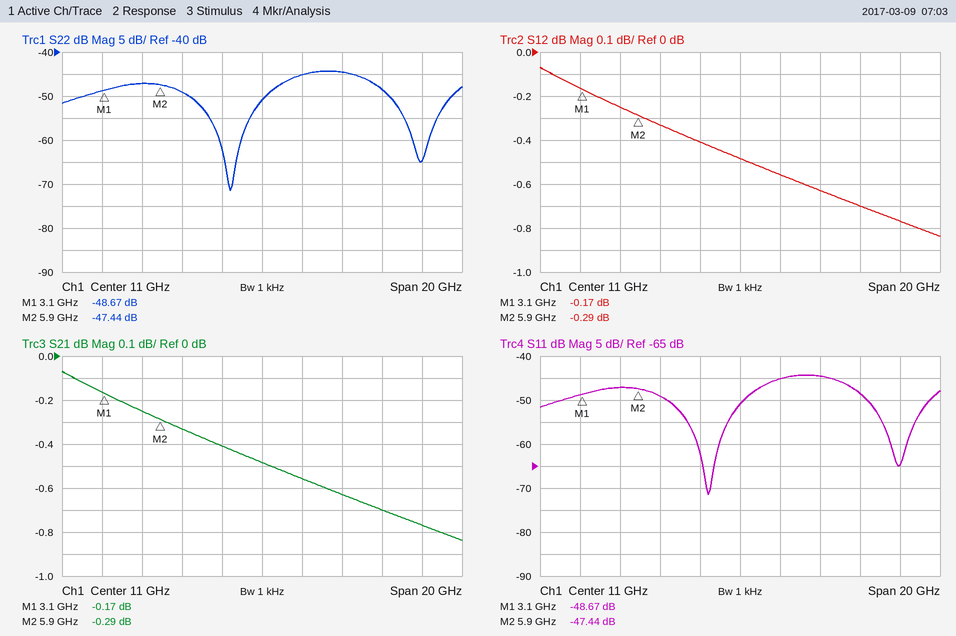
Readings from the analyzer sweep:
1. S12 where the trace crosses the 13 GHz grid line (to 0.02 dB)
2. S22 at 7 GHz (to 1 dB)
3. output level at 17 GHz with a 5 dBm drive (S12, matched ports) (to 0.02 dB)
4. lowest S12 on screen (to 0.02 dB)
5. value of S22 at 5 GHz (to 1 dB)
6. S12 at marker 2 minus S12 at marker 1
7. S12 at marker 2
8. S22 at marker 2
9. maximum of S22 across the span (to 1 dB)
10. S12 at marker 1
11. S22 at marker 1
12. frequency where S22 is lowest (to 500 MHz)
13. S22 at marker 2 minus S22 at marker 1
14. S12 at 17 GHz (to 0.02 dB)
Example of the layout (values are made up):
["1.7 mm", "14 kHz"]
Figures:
["-0.56 dB", "-49 dB", "4.30 dBm", "-0.84 dB", "-47 dB", "-0.12 dB", "-0.29 dB", "-47.44 dB", "-44 dB", "-0.17 dB", "-48.67 dB", "9.5 GHz", "1.23 dB", "-0.70 dB"]
